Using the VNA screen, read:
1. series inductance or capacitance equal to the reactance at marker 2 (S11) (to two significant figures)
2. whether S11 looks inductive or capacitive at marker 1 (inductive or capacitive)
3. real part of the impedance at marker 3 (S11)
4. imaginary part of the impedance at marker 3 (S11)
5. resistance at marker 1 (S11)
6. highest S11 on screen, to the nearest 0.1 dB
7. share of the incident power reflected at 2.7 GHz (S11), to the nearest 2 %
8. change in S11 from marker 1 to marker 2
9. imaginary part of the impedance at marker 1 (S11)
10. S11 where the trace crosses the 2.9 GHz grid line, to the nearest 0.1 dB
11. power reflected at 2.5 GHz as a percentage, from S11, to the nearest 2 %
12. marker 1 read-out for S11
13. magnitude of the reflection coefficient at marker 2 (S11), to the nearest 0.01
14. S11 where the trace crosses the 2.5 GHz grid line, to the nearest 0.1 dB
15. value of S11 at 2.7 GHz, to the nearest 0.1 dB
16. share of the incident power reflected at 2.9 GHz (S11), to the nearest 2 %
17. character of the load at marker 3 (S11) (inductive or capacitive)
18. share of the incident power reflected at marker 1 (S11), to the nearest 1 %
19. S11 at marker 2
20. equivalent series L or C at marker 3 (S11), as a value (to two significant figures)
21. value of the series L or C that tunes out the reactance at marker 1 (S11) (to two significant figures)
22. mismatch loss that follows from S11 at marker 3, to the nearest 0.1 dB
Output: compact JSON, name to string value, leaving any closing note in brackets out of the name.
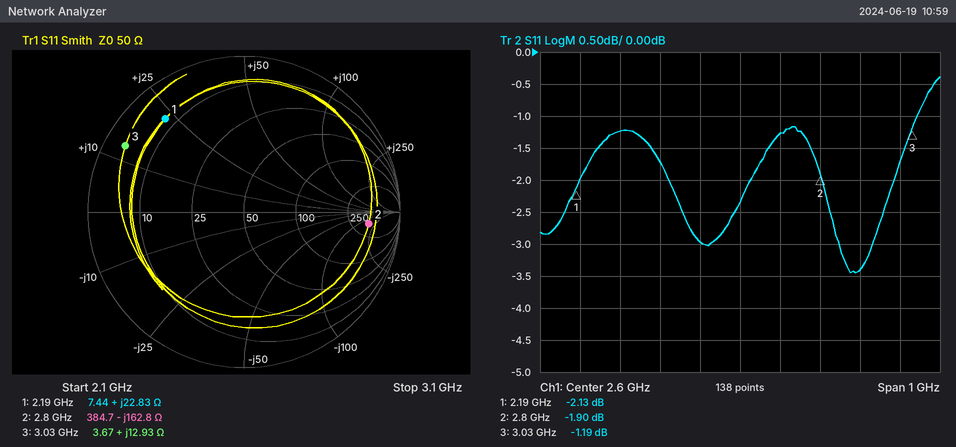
{"series inductance or capacitance equal to the reactance at marker 2 (S11)": "350 fF", "whether S11 looks inductive or capacitive at marker 1": "inductive", "real part of the impedance at marker 3": "3.67 Ω", "imaginary part of the impedance at marker 3": "+12.93 Ω", "resistance at marker 1": "7.44 Ω", "highest S11 on screen, to the nearest 0.1 dB": "-0.4 dB", "share of the incident power reflected at 2.7 GHz (S11), to the nearest 2 %": "74 %", "change in S11 from marker 1 to marker 2": "0.23 dB", "imaginary part of the impedance at marker 1": "+22.83 Ω", "S11 where the trace crosses the 2.9 GHz grid line, to the nearest 0.1 dB": "-3.4 dB", "power reflected at 2.5 GHz as a percentage, from S11, to the nearest 2 %": "50 %", "marker 1 read-out for S11": "-2.13 dB", "magnitude of the reflection coefficient at marker 2 (S11), to the nearest 0.01": "0.80", "S11 where the trace crosses the 2.5 GHz grid line, to the nearest 0.1 dB": "-3.0 dB", "value of S11 at 2.7 GHz, to the nearest 0.1 dB": "-1.3 dB", "share of the incident power reflected at 2.9 GHz (S11), to the nearest 2 %": "46 %", "character of the load at marker 3 (S11)": "inductive", "share of the incident power reflected at marker 1 (S11), to the nearest 1 %": "61 %", "S11 at marker 2": "-1.90 dB", "equivalent series L or C at marker 3 (S11), as a value": "680 pH", "value of the series L or C that tunes out the reactance at marker 1 (S11)": "3.2 pF", "mismatch loss that follows from S11 at marker 3, to the nearest 0.1 dB": "6.2 dB"}
